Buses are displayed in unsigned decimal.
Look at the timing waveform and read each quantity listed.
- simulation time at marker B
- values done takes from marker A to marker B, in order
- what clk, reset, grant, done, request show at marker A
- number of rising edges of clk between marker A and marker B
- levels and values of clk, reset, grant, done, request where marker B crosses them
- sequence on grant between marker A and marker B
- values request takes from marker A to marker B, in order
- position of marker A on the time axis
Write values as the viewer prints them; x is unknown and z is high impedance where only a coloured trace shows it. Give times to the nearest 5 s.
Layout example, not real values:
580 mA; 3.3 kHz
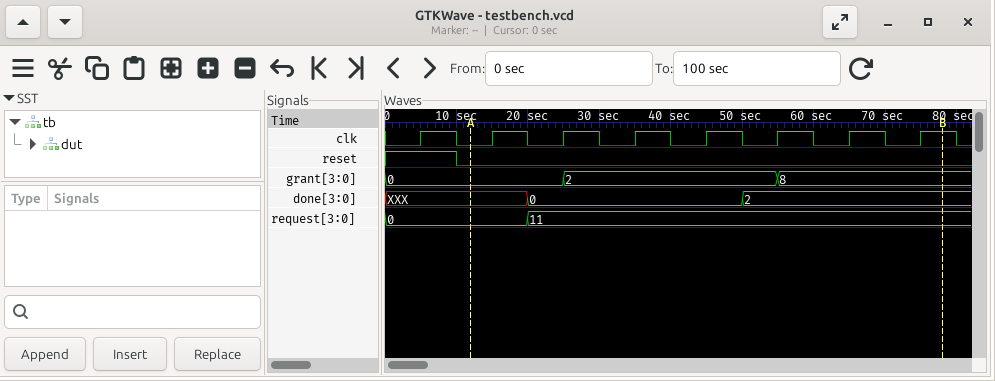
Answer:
80 s; XXX, 0, 2; clk=0, reset=0, grant=0, done=XXX, request=0; 7; clk=1, reset=0, grant=8, done=2, request=11; 0, 2, 8; 0, 11; 10 s
